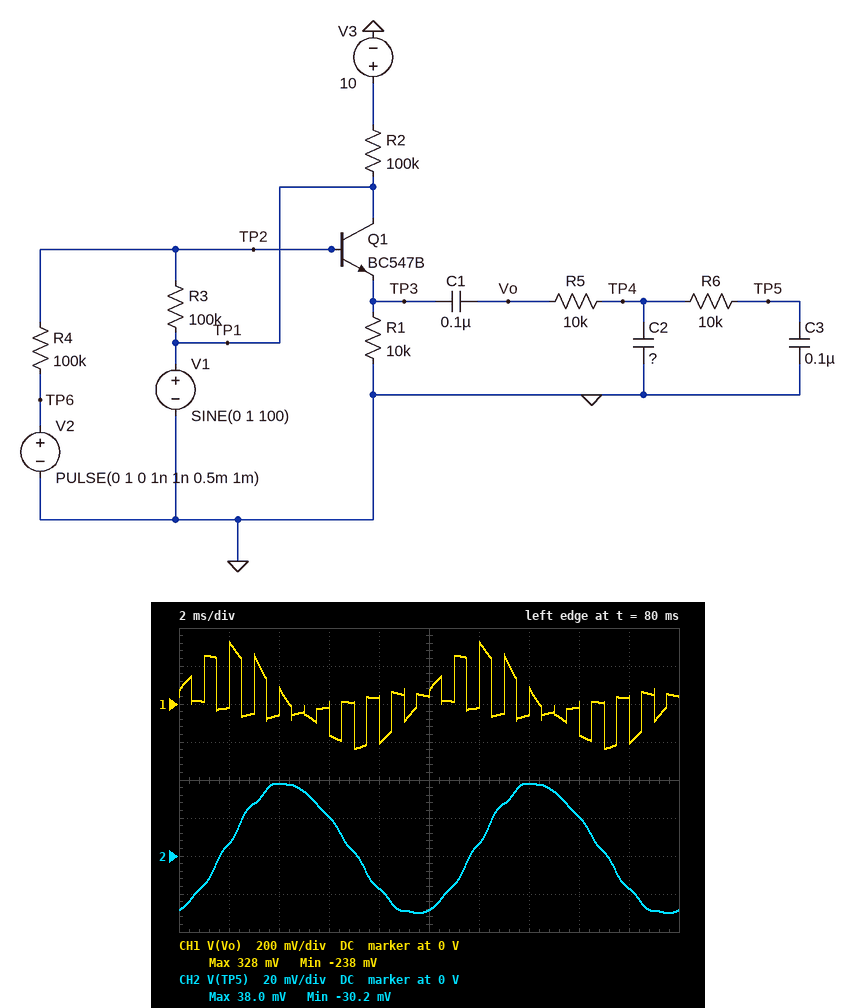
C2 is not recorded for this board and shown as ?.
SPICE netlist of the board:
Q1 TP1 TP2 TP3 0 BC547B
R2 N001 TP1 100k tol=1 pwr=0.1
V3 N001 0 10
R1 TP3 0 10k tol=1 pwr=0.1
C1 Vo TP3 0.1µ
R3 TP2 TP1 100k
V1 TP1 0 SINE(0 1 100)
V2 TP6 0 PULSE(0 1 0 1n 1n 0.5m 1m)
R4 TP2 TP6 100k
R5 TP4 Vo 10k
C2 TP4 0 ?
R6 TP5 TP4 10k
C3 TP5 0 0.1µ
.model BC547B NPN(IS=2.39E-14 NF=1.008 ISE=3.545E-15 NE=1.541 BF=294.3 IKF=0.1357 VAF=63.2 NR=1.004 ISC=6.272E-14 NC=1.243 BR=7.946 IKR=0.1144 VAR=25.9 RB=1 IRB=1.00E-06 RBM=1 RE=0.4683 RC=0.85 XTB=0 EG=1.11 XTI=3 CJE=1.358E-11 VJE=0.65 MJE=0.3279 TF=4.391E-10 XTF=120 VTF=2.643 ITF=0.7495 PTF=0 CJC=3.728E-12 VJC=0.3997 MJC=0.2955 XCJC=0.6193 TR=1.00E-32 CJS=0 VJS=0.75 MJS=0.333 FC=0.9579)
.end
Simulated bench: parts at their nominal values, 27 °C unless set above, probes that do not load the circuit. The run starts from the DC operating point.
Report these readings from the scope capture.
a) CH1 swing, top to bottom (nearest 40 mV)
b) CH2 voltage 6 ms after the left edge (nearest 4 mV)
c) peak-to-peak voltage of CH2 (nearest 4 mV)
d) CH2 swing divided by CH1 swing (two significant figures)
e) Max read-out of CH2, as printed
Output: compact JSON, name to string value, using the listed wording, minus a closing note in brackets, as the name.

{"CH1 swing, top to bottom": "560 mV", "CH2 voltage 6 ms after the left edge": "20 mV", "peak-to-peak voltage of CH2": "68 mV", "CH2 swing divided by CH1 swing": "0.12", "Max read-out of CH2, as printed": "38.0 mV"}
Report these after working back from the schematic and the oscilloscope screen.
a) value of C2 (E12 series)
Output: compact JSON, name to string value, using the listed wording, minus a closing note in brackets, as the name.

{"value of C2": "330 nF"}
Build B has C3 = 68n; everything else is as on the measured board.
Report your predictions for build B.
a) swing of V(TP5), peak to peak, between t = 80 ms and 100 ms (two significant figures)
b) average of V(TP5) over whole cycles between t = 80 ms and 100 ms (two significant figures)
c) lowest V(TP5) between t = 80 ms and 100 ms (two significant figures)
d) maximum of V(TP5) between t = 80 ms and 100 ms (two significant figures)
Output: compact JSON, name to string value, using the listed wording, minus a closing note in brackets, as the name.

{"swing of V(TP5), peak to peak, between t = 80 ms and 100 ms": "78 mV", "average of V(TP5) over whole cycles between t = 80 ms and 100 ms": "4.1 mV", "lowest V(TP5) between t = 80 ms and 100 ms": "-34 mV", "maximum of V(TP5) between t = 80 ms and 100 ms": "44 mV"}
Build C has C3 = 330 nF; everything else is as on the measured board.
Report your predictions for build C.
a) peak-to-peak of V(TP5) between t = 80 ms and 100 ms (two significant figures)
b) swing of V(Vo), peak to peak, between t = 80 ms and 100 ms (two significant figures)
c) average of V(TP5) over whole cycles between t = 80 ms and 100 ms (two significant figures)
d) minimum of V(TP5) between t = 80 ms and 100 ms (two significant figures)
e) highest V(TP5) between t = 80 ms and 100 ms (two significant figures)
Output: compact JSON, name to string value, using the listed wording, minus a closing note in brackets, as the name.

{"peak-to-peak of V(TP5) between t = 80 ms and 100 ms": "34 mV", "swing of V(Vo), peak to peak, between t = 80 ms and 100 ms": "580 mV", "average of V(TP5) over whole cycles between t = 80 ms and 100 ms": "2.7 mV", "minimum of V(TP5) between t = 80 ms and 100 ms": "-14 mV", "highest V(TP5) between t = 80 ms and 100 ms": "19 mV"}
